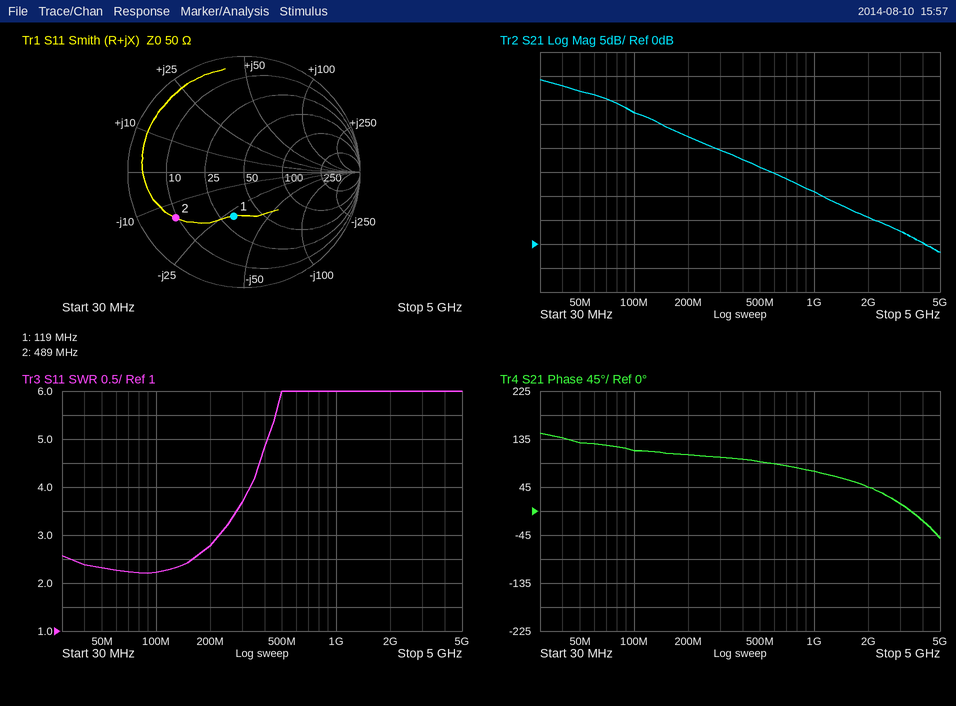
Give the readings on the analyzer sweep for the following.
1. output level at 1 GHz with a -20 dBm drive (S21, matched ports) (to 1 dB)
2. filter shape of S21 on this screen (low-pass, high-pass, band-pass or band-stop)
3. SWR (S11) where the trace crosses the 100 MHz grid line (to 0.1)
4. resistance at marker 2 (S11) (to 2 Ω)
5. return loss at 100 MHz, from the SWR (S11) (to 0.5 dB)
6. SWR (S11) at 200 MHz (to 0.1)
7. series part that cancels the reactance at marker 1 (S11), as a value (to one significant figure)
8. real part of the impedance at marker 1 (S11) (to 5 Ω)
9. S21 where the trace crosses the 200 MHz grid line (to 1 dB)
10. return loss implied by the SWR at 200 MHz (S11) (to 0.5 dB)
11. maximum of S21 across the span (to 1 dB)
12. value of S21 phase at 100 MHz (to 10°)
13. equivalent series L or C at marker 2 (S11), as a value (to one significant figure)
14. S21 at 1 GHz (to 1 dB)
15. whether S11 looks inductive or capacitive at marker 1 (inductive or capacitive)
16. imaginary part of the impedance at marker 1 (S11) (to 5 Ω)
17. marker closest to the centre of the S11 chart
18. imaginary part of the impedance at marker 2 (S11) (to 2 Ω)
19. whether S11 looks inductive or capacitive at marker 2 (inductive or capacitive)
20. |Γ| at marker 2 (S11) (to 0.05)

-9 dBm
low-pass
2.2
10 Ω
8.5 dB
2.8
40 nH
30 Ω
22 dB
6.5 dB
34 dB
110°
20 pF
11 dB
capacitive
-30 Ω
marker 1
-14 Ω
capacitive
0.70
